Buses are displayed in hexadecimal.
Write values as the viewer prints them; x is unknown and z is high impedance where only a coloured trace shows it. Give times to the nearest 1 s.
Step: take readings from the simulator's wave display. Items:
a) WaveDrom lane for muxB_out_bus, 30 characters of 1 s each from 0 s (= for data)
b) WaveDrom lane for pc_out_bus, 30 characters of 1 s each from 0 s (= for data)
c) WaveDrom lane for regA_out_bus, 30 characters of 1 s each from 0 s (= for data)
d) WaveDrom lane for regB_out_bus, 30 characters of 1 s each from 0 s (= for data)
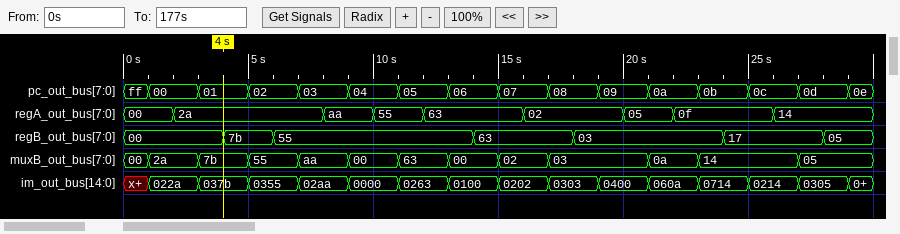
{name: 'muxB_out_bus', wave: '==.=.=.=.=.=.=.=.=...=.=...=..', data: '00 2a 7b 55 aa 00 63 00 02 03 0a 14 05'}
{name: 'pc_out_bus', wave: '==.=.=.=.=.=.=.=.=.=.=.=.=.=.=', data: 'ff 00 01 02 03 04 05 06 07 08 09 0a 0b 0c 0d 0e'}
{name: 'regA_out_bus', wave: '=.=.....=.=.=...=...=.=...=...', data: '00 2a aa 55 63 02 05 0f 14'}
{name: 'regB_out_bus', wave: '=...=.=.......=...=.....=...=.', data: '00 7b 55 63 03 17 05'}
